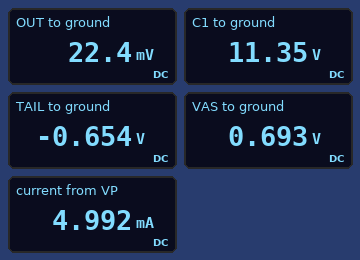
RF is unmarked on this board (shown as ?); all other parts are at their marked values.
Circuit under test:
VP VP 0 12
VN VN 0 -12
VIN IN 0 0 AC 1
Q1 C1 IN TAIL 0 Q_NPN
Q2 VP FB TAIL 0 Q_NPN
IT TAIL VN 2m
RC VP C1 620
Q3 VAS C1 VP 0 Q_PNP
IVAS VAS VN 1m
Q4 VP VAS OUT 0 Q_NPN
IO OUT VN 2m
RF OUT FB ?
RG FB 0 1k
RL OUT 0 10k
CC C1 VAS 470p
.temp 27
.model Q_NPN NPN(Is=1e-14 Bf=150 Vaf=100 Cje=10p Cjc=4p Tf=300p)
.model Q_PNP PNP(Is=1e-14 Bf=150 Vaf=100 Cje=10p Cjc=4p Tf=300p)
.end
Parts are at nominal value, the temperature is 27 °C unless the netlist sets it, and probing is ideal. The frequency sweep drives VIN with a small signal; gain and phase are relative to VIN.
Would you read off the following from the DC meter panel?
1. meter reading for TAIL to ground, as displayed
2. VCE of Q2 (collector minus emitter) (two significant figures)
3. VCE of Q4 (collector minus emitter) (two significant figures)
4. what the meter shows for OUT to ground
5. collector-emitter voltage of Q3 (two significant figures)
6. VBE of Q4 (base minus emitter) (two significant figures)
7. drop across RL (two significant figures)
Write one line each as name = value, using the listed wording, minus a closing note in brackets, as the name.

meter reading for TAIL to ground, as displayed = -0.654 V
VCE of Q2 (collector minus emitter) = 13 V
VCE of Q4 (collector minus emitter) = 12 V
what the meter shows for OUT to ground = 22.4 mV
collector-emitter voltage of Q3 = -11 V
VBE of Q4 (base minus emitter) = 670 mV
drop across RL = 22 mV
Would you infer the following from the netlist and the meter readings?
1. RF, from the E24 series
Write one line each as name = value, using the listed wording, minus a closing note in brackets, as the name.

RF, from the E24 series = 13 kΩ
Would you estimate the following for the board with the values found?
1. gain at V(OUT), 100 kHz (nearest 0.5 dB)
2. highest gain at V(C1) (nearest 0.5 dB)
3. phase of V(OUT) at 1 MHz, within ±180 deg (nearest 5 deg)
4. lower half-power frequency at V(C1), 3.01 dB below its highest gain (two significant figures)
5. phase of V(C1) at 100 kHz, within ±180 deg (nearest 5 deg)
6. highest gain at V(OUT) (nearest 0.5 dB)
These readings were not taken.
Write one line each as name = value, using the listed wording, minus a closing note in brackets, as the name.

gain at V(OUT), 100 kHz = 22.5 dB
highest gain at V(C1) = -7.0 dB
phase of V(OUT) at 1 MHz, within ±180 deg = -75 deg
lower half-power frequency at V(C1), 3.01 dB below its highest gain = 400 kHz
phase of V(C1) at 100 kHz, within ±180 deg = -105 deg
highest gain at V(OUT) = 23.0 dB
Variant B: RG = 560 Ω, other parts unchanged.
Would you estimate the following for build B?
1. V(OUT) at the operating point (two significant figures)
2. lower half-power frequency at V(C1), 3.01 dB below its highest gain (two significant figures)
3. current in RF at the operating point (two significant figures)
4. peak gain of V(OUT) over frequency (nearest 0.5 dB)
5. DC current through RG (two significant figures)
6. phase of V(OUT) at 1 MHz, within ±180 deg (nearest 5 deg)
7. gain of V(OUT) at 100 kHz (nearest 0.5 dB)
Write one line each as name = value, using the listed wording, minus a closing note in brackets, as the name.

V(OUT) at the operating point = -14 mV
lower half-power frequency at V(C1), 3.01 dB below its highest gain = 240 kHz
current in RF at the operating point = 780 nA
peak gain of V(OUT) over frequency = 27.5 dB
DC current through RG = 6.3 µA
phase of V(OUT) at 1 MHz, within ±180 deg = -85 deg
gain of V(OUT) at 100 kHz = 27.0 dB
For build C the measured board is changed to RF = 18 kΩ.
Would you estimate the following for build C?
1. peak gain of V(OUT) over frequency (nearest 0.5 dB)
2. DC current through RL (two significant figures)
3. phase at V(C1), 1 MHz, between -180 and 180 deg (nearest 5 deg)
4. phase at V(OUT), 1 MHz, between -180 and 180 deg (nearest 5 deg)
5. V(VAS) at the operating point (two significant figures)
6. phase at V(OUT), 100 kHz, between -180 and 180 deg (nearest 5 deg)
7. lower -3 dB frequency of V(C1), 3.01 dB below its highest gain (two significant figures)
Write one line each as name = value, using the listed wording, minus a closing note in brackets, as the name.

peak gain of V(OUT) over frequency = 25.5 dB
DC current through RL = 3.2 µA
phase at V(C1), 1 MHz, between -180 and 180 deg = -170 deg
phase at V(OUT), 1 MHz, between -180 and 180 deg = -80 deg
V(VAS) at the operating point = 700 mV
phase at V(OUT), 100 kHz, between -180 and 180 deg = -20 deg
lower -3 dB frequency of V(C1), 3.01 dB below its highest gain = 290 kHz
